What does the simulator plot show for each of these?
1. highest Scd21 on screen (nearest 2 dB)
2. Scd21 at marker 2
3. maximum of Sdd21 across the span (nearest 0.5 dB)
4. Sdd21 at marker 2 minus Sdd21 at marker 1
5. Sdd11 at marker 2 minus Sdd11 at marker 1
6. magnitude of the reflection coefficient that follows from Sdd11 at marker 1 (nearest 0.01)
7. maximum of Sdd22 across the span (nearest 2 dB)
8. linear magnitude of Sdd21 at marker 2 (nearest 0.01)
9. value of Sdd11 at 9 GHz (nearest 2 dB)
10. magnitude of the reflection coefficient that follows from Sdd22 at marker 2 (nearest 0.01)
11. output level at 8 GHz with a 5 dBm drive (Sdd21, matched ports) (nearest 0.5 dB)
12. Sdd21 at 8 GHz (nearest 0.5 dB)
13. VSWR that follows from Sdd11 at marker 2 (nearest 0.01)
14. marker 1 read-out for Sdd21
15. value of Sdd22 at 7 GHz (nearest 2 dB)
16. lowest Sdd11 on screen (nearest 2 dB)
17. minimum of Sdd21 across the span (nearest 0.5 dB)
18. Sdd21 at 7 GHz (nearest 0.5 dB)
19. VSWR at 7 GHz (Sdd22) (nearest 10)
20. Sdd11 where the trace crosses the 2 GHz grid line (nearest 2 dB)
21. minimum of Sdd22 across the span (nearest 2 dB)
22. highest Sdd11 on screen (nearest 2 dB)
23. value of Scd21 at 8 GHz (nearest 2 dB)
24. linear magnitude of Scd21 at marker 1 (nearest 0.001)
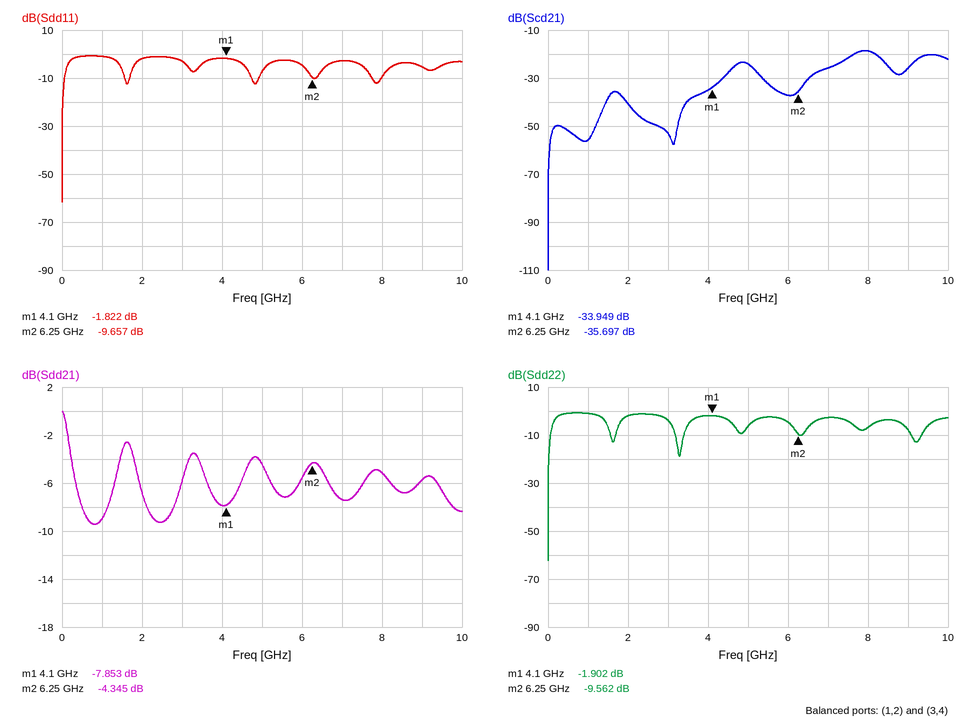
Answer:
-18 dB
-35.697 dB
0.0 dB
3.508 dB
-7.835 dB
0.81
0 dB
0.61
-6 dB
0.33
0.0 dBm
-5.0 dB
1.98
-7.853 dB
-2 dB
-62 dB
-9.5 dB
-7.5 dB
10
-2 dB
-62 dB
0 dB
-18 dB
0.020
